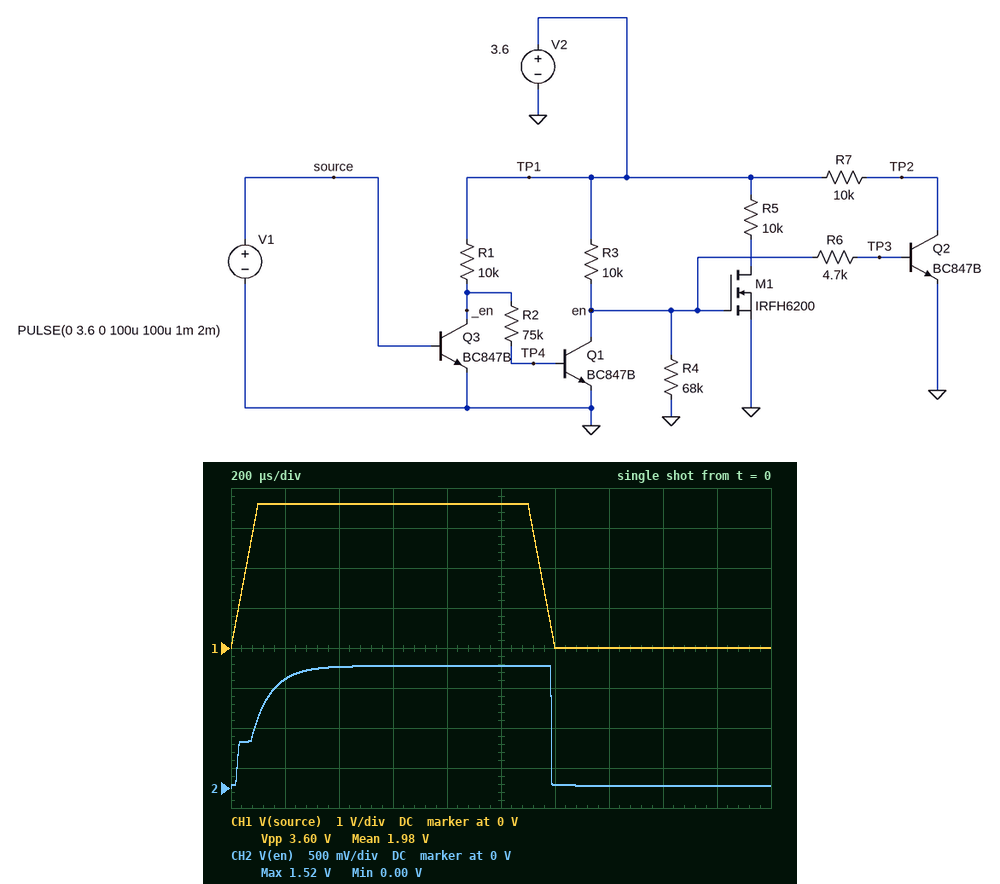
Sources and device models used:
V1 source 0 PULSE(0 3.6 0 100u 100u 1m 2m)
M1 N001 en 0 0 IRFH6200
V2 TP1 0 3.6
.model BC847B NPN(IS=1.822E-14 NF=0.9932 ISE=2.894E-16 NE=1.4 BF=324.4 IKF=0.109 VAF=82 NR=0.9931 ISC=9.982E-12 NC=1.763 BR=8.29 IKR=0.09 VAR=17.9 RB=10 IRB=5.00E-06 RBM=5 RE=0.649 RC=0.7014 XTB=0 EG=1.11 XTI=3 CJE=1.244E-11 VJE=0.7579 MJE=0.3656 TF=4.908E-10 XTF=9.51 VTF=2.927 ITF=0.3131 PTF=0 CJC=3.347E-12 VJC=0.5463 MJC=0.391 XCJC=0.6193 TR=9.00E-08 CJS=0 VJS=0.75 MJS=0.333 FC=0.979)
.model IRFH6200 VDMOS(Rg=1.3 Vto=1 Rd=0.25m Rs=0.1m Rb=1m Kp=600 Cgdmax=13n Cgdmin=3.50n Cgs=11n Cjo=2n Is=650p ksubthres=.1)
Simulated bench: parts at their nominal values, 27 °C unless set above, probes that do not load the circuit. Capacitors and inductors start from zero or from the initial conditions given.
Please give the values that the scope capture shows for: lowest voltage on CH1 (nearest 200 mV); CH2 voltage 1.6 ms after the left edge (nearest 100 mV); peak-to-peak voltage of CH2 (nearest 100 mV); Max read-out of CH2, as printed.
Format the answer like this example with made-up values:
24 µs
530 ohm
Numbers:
0 V
0 V
1.5 V
1.52 V
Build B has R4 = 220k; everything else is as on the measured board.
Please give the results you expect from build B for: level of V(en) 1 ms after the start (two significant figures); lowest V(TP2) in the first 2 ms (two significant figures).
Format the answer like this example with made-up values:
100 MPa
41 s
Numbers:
1.6 V
9.4 mV
